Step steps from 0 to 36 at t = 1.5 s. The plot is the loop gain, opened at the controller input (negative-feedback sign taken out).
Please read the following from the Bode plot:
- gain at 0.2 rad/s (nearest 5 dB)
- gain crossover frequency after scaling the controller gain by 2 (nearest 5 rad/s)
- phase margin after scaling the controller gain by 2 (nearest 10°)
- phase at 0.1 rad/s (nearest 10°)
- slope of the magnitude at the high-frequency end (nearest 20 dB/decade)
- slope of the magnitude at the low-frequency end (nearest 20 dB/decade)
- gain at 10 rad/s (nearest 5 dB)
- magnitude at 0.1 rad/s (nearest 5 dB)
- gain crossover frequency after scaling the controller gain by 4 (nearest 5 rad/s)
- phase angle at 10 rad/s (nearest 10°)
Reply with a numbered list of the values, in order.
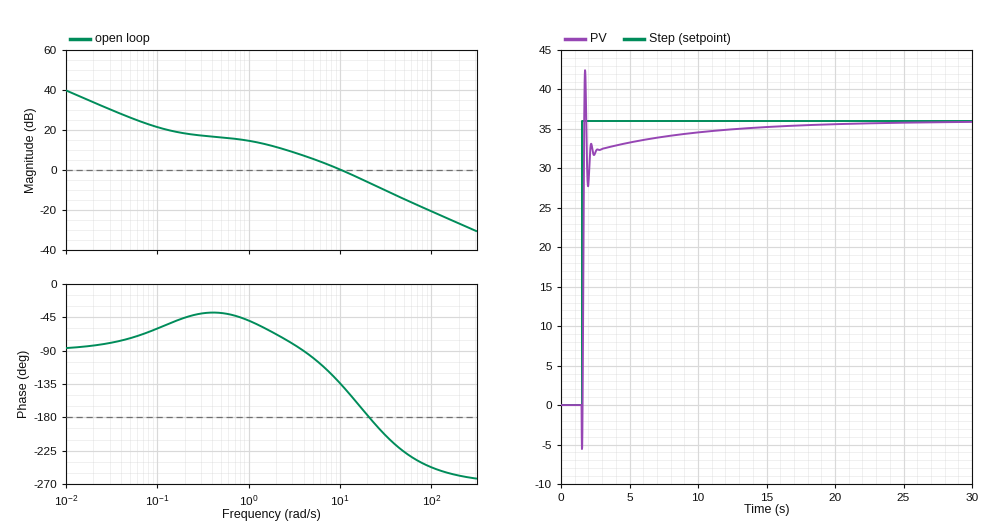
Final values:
1. 20 dB
2. 20 rad/s
3. 0°
4. -60°
5. -20 dB/decade
6. -20 dB/decade
7. 0 dB
8. 20 dB
9. 40 rad/s
10. -130°
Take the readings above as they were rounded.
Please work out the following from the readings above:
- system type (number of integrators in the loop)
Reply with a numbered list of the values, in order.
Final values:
1. 1
